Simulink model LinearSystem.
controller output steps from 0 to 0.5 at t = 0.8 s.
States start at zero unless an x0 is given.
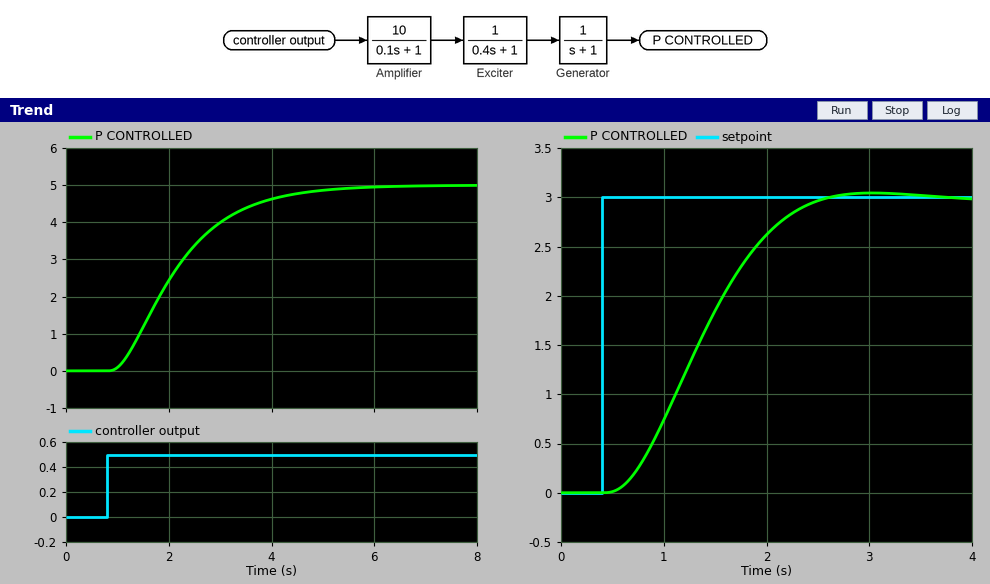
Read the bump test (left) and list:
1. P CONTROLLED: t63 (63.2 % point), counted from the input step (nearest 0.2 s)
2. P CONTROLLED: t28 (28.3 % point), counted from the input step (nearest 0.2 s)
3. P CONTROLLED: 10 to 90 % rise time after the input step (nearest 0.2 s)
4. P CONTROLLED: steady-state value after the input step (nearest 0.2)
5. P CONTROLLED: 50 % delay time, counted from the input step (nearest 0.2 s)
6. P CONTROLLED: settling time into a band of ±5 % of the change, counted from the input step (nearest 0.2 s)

1.6 s
0.8 s
2.4 s
5.0
1.2 s
3.6 s
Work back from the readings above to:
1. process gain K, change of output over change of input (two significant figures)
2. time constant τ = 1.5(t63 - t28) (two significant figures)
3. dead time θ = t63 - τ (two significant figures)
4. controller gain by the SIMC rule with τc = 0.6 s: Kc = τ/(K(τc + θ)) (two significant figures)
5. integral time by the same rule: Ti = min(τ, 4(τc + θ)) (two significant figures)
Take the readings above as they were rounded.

10
1.2 s
0.40 s
0.12
1.2 s
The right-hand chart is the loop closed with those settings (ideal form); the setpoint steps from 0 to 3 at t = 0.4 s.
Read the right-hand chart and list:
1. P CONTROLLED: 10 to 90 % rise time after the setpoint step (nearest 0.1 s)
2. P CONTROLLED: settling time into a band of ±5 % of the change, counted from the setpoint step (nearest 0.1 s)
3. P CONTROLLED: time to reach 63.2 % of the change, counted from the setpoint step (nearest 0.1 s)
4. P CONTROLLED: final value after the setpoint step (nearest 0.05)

1.3 s
1.9 s
1.1 s
3.00
